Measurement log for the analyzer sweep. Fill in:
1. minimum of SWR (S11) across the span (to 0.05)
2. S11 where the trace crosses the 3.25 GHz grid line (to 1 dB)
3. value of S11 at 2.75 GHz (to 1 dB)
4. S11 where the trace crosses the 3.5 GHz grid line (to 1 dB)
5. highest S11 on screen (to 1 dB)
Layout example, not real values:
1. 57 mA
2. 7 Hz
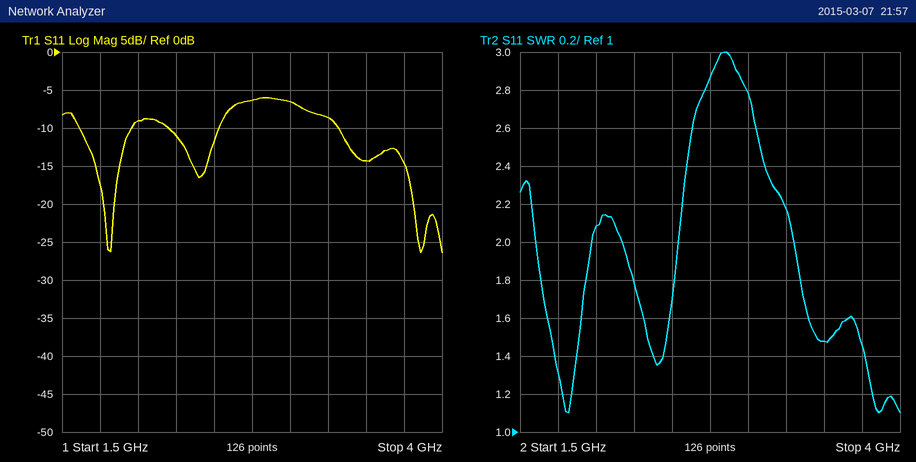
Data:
1. 1.10
2. -9 dB
3. -6 dB
4. -14 dB
5. -6 dB
